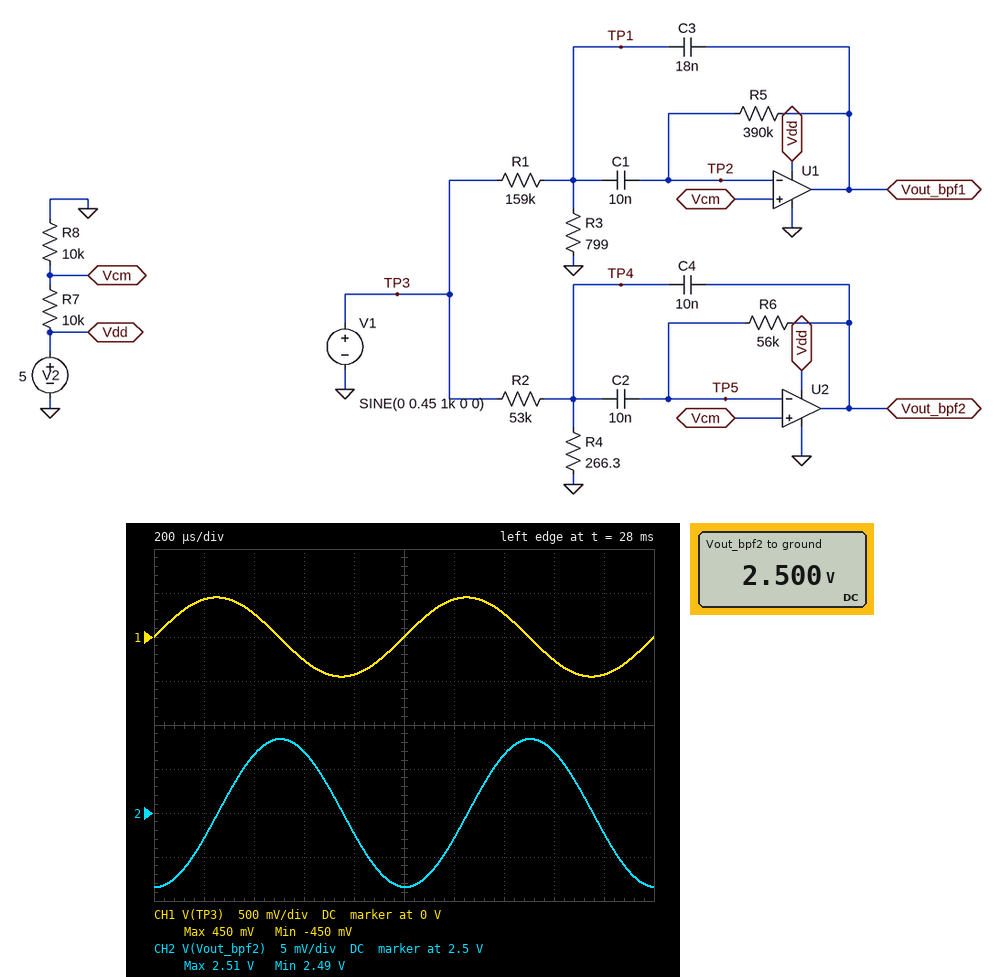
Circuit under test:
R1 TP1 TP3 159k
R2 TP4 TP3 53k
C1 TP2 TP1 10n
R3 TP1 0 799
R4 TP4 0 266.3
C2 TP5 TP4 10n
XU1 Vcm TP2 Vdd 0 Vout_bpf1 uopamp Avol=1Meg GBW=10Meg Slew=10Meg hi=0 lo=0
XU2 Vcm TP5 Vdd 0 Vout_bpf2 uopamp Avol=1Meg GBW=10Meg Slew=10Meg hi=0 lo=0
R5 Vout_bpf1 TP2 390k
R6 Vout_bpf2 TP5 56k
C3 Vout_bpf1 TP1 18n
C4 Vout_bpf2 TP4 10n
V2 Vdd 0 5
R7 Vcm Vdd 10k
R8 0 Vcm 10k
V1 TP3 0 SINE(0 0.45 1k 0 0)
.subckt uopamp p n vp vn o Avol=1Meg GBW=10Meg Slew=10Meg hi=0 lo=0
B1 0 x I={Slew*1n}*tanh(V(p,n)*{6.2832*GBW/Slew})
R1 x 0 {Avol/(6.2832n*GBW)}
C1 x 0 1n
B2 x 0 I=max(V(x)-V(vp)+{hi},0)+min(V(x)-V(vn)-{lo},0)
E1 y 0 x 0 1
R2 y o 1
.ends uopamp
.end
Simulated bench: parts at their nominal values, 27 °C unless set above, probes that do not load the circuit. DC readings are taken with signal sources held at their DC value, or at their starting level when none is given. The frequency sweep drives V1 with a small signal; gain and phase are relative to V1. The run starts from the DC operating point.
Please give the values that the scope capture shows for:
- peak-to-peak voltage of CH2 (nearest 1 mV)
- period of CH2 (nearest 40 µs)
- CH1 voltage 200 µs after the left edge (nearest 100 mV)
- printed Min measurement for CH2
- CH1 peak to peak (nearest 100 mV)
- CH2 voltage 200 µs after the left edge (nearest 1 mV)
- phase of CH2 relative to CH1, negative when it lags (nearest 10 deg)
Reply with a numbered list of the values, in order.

1. 17 mV
2. 1.00 ms
3. 400 mV
4. 2.49 V
5. 900 mV
6. 2.497 V
7. -90 deg
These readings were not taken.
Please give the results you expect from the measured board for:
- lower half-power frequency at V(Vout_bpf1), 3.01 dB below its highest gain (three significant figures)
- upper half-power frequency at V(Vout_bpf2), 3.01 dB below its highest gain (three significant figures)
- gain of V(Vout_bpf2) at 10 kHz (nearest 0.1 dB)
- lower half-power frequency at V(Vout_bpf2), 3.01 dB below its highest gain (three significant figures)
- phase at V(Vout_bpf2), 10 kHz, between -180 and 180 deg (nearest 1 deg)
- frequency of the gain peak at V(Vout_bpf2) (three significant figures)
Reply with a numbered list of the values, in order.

1. 642 Hz
2. 4.41 kHz
3. -28.9 dB
4. 3.85 kHz
5. 94 deg
6. 4.12 kHz
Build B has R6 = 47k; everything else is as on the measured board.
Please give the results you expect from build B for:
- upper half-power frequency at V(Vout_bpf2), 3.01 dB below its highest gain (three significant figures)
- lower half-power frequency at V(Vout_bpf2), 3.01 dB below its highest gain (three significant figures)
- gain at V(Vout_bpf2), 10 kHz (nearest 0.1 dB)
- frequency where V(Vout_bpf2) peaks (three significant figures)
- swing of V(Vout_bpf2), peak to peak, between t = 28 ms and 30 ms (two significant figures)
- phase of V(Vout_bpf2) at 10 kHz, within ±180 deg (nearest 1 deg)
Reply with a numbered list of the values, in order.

1. 4.85 kHz
2. 4.17 kHz
3. -28.6 dB
4. 4.50 kHz
5. 14 mV
6. 95 deg
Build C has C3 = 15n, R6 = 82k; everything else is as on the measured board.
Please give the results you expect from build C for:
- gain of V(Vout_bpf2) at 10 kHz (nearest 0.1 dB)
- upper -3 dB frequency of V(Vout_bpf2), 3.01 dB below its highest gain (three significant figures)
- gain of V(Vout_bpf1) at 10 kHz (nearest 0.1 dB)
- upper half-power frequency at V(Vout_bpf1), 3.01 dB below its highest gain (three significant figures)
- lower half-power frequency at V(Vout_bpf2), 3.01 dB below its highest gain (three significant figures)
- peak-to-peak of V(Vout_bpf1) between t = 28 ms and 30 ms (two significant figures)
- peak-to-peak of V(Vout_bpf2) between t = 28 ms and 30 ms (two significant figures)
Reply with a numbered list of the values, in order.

1. -29.4 dB
2. 3.60 kHz
3. -43.5 dB
4. 772 Hz
5. 3.22 kHz
6. 130 mV
7. 25 mV
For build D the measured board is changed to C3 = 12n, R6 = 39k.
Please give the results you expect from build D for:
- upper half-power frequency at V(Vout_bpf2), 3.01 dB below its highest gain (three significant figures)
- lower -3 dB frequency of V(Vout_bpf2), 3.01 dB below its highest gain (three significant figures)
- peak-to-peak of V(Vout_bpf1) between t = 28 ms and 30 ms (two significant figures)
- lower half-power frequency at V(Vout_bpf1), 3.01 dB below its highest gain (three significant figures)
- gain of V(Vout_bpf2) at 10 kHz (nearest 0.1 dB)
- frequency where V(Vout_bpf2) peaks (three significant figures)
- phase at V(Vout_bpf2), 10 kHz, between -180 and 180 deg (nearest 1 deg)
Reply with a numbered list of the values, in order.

1. 5.36 kHz
2. 4.55 kHz
3. 230 mV
4. 788 Hz
5. -28.1 dB
6. 4.94 kHz
7. 96 deg
